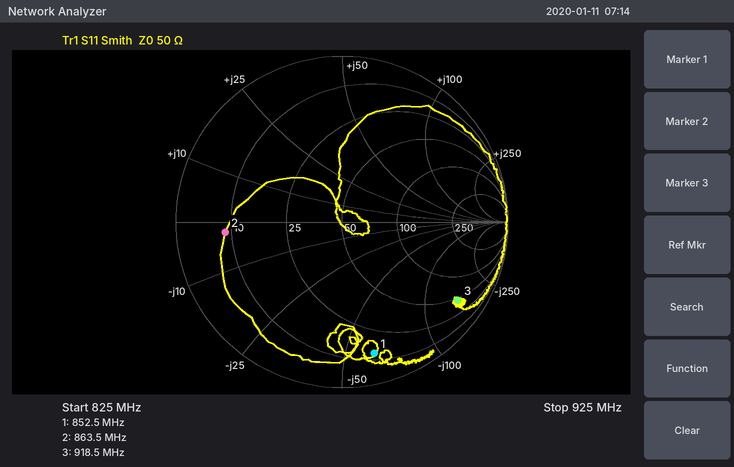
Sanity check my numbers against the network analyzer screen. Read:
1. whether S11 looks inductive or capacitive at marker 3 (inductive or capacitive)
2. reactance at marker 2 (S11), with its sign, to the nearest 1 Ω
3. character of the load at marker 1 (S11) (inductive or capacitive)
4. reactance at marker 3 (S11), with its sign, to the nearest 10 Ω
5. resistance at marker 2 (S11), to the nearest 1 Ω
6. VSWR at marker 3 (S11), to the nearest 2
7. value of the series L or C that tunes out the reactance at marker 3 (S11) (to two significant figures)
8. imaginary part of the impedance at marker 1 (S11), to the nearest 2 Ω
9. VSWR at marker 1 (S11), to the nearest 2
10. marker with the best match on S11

capacitive
-2 Ω
capacitive
-150 Ω
9 Ω
12
26 nH
-62 Ω
10
marker 2
